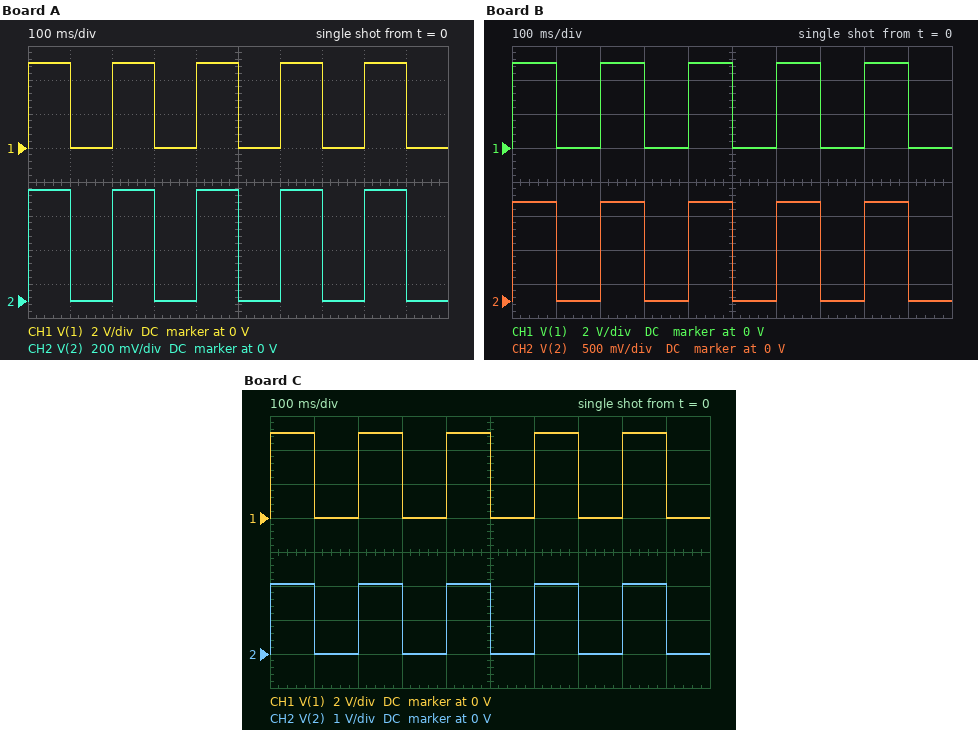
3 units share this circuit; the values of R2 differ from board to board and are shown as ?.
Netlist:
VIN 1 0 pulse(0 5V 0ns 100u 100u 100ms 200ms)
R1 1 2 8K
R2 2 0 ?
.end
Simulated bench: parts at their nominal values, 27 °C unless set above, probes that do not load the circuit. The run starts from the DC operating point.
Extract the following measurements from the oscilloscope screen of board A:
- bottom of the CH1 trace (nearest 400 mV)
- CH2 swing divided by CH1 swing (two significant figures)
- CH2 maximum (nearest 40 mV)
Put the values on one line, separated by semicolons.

0 V; 0.13; 640 mV
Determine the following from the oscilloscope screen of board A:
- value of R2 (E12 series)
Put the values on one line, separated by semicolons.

1.2 kΩ
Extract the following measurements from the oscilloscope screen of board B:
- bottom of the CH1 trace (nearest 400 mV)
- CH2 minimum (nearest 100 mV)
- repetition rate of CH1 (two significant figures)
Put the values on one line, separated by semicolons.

0 V; 0 V; 5.0 Hz
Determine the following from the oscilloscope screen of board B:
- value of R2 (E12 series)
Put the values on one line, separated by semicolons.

3.3 kΩ
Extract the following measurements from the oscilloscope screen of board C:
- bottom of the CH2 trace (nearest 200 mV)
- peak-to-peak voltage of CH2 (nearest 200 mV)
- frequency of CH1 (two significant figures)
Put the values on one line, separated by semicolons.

0 V; 2.0 V; 5.0 Hz
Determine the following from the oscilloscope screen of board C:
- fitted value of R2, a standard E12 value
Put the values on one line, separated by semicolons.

5.6 kΩ
